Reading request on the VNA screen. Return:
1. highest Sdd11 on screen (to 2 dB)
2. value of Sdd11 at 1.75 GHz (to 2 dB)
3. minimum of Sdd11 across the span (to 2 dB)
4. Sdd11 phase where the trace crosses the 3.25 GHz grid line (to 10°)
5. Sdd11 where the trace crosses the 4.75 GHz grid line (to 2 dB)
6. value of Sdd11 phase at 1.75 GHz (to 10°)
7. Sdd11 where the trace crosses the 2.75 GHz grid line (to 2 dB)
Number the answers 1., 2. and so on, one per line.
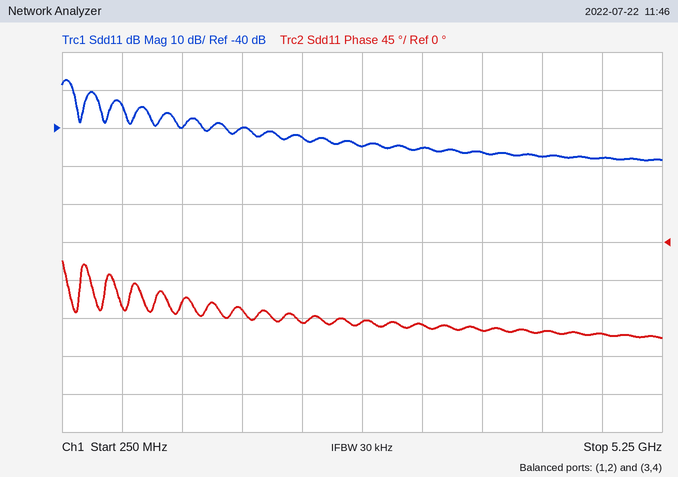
1. -28 dB
2. -40 dB
3. -48 dB
4. -100°
5. -48 dB
6. -80°
7. -44 dB
